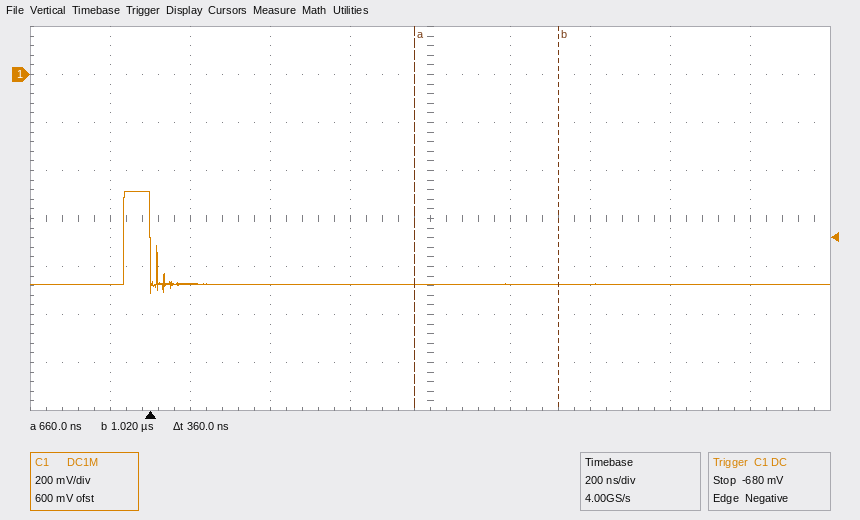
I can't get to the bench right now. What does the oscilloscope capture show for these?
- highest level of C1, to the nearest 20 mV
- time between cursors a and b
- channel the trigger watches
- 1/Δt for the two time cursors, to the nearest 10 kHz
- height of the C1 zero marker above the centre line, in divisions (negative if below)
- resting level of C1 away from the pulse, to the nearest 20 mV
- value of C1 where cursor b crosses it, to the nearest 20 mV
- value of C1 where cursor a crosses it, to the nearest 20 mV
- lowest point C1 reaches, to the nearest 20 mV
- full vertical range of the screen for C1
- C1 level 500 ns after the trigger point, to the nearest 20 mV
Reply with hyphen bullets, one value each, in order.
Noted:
- -480 mV
- 360 ns
- C1
- 2.78 MHz
- +3.0 div
- -880 mV
- -880 mV
- -880 mV
- -920 mV
- 1.6 V
- -880 mV
